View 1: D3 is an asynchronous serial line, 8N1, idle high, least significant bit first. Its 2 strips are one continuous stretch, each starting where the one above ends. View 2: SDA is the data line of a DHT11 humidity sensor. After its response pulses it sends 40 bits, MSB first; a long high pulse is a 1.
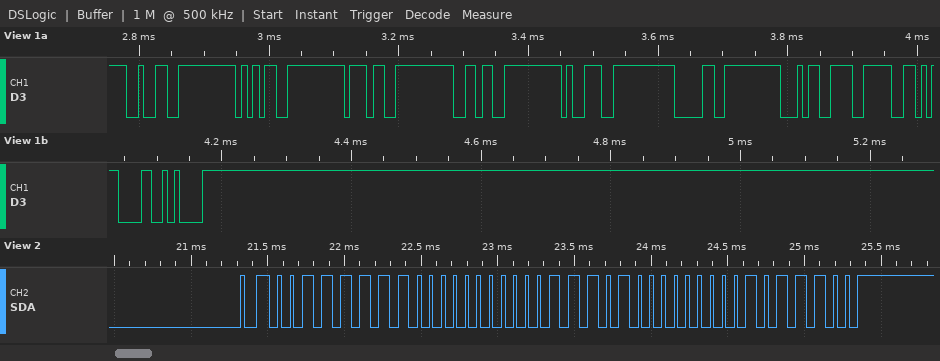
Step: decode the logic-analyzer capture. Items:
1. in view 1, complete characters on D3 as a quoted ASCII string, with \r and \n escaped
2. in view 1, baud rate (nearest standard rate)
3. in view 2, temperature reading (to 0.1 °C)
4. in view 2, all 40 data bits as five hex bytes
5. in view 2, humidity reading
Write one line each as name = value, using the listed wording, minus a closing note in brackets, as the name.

in view 1, complete characters on D3 as a quoted ASCII string, with \r and \n escaped = "2576904>\r\n"
in view 1, baud rate = 115200 baud
in view 2, temperature reading = 29.0 °C
in view 2, all 40 data bits as five hex bytes = 3F 00 1D 00 5C
in view 2, humidity reading = 63 %
